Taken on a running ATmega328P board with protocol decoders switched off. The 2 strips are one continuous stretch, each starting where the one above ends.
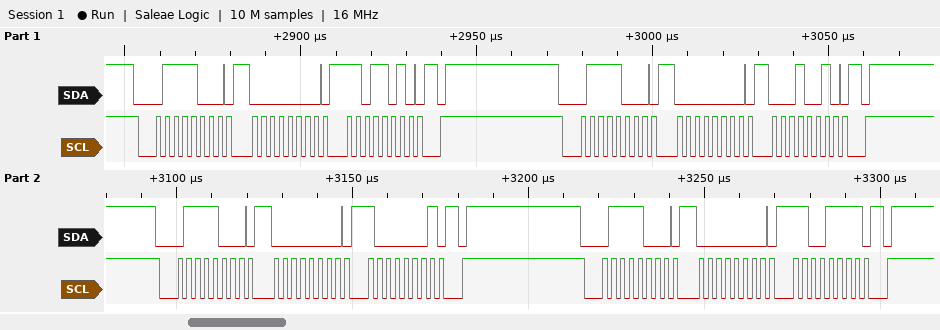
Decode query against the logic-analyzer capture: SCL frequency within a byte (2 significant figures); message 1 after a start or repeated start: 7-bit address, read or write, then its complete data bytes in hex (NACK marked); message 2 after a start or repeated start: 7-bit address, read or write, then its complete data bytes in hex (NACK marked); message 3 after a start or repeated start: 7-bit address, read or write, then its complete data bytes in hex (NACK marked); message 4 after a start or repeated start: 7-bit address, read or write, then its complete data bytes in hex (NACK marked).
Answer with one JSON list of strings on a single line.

["400 kHz", "0x3C write: 00 DA", "0x3C write: 00 12", "0x3C write: 00 81", "0x3C write: 00 CF"]
